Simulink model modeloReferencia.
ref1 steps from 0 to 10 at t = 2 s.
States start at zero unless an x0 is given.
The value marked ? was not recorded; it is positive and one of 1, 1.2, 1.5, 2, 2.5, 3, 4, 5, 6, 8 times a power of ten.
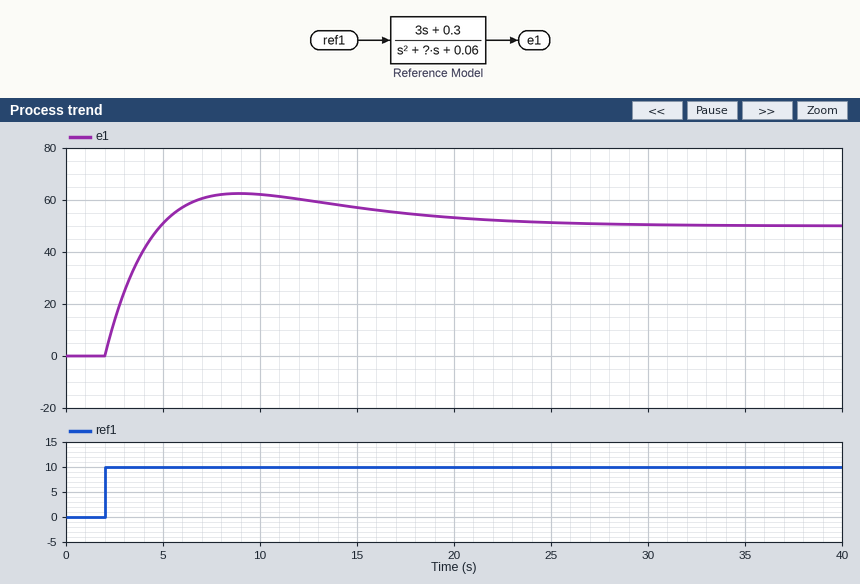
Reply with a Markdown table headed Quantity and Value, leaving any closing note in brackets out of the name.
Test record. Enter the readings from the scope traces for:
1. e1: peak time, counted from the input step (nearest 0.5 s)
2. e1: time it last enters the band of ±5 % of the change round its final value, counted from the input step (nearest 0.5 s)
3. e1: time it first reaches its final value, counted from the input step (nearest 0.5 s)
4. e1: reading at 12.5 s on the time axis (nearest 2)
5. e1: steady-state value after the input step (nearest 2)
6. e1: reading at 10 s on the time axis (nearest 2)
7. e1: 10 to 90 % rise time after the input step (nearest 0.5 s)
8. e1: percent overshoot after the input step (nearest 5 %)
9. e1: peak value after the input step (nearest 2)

| Quantity | Value |
|---|---|
| e1: peak time, counted from the input step | 7.0 s |
| e1: time it last enters the band of ±5 % of the change round its final value, counted from the input step | 19.5 s |
| e1: time it first reaches its final value, counted from the input step | 3.0 s |
| e1: reading at 12.5 s on the time axis | 60 |
| e1: steady-state value after the input step | 50 |
| e1: reading at 10 s on the time axis | 62 |
| e1: 10 to 90 % rise time after the input step | 2.0 s |
| e1: percent overshoot after the input step | 25 % |
| e1: peak value after the input step | 62 |
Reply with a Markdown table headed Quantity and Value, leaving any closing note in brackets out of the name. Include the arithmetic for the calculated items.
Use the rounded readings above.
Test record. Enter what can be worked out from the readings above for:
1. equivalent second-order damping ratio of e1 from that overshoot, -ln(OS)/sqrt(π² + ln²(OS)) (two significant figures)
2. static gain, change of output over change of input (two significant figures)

| Quantity | Value |
|---|---|
| equivalent second-order damping ratio of e1 from that overshoot, -ln(OS)/sqrt(π² + ln²(OS)) | ln(0.25) = -1.386; 1.386 / sqrt(9.870 + 1.922) = 0.40 |
| static gain, change of output over change of input | (50 - 0) / (10 - 0) = 5.0 |
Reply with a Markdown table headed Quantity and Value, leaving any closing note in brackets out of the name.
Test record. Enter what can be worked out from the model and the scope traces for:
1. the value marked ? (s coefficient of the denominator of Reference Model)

| Quantity | Value |
|---|---|
| the value marked ? | 0.5 |
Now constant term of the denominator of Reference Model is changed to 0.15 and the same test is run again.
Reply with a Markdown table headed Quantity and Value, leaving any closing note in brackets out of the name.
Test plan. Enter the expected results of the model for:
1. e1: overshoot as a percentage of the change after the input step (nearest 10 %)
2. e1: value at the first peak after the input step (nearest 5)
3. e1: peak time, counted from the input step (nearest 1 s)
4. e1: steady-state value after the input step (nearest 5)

| Quantity | Value |
|---|---|
| e1: overshoot as a percentage of the change after the input step | 130 % |
| e1: value at the first peak after the input step | 45 |
| e1: peak time, counted from the input step | 4 s |
| e1: steady-state value after the input step | 20 |
